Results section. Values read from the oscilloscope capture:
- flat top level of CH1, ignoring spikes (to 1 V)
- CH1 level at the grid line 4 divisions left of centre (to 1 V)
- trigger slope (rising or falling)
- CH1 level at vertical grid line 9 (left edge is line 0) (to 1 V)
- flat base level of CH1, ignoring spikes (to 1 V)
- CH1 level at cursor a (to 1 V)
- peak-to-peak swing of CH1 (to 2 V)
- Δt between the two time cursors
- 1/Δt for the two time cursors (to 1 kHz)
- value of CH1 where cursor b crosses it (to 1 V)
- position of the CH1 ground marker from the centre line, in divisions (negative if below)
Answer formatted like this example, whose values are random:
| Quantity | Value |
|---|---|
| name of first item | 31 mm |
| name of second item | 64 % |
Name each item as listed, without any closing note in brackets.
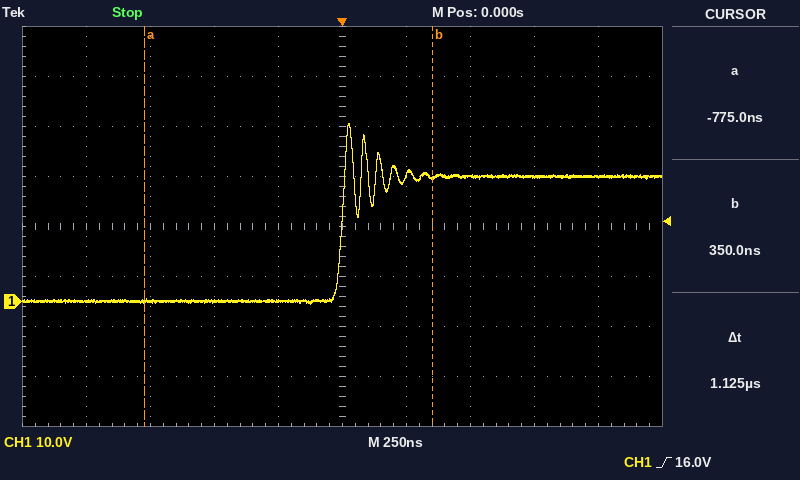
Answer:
| Quantity | Value |
|---|---|
| flat top level of CH1, ignoring spikes | 25 V |
| CH1 level at the grid line 4 divisions left of centre | 0 V |
| trigger slope | rising |
| CH1 level at vertical grid line 9 (left edge is line 0) | 25 V |
| flat base level of CH1, ignoring spikes | 0 V |
| CH1 level at cursor a | 0 V |
| peak-to-peak swing of CH1 | 36 V |
| Δt between the two time cursors | 1.125 µs |
| 1/Δt for the two time cursors | 889 kHz |
| value of CH1 where cursor b crosses it | 25 V |
| position of the CH1 ground marker from the centre line, in divisions | -1.5 div |
